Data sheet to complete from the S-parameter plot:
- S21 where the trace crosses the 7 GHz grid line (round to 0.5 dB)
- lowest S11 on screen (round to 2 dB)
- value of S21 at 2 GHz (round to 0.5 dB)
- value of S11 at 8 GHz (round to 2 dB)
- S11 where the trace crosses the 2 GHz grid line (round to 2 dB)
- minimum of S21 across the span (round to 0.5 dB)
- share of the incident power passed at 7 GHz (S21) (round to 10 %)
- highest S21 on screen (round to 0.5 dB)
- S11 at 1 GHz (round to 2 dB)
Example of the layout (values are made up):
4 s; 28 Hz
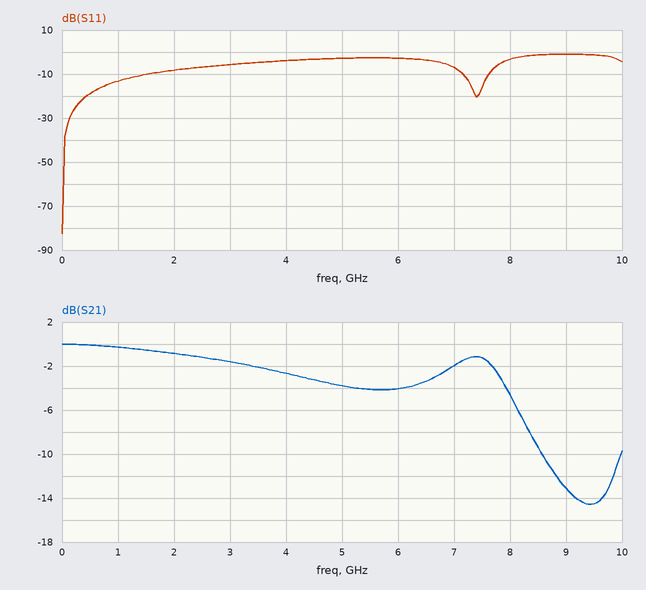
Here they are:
-2.0 dB; -82 dB; -1.0 dB; -4 dB; -8 dB; -14.5 dB; 60 %; 0.0 dB; -14 dB
